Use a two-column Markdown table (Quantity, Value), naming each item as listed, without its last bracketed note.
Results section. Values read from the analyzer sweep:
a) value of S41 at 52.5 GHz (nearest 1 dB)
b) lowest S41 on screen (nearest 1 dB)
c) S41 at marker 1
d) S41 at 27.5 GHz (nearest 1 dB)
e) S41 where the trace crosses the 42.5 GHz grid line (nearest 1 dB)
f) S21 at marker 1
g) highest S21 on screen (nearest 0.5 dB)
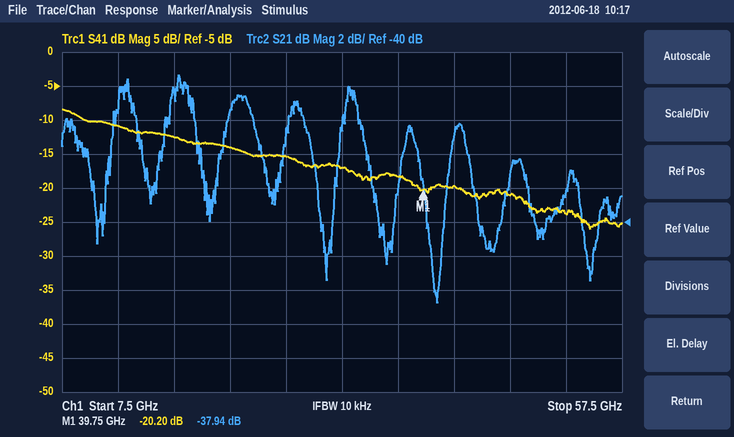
| Quantity | Value |
|---|---|
| value of S41 at 52.5 GHz | -24 dB |
| lowest S41 on screen | -26 dB |
| S41 at marker 1 | -20.20 dB |
| S41 at 27.5 GHz | -15 dB |
| S41 where the trace crosses the 42.5 GHz grid line | -20 dB |
| S21 at marker 1 | -37.94 dB |
| highest S21 on screen | -31.5 dB |
